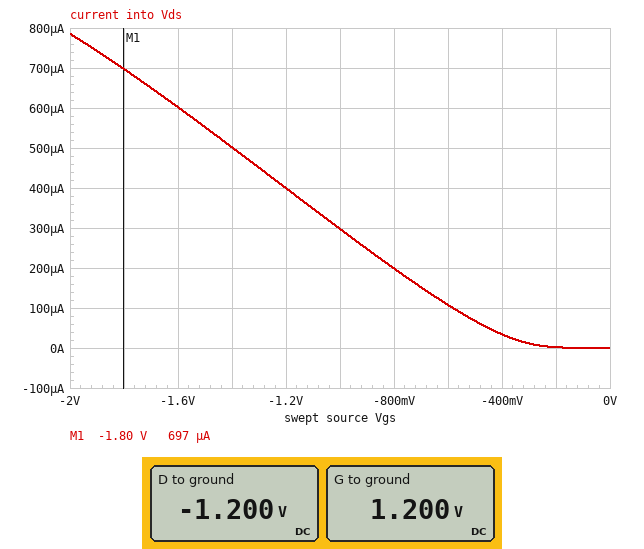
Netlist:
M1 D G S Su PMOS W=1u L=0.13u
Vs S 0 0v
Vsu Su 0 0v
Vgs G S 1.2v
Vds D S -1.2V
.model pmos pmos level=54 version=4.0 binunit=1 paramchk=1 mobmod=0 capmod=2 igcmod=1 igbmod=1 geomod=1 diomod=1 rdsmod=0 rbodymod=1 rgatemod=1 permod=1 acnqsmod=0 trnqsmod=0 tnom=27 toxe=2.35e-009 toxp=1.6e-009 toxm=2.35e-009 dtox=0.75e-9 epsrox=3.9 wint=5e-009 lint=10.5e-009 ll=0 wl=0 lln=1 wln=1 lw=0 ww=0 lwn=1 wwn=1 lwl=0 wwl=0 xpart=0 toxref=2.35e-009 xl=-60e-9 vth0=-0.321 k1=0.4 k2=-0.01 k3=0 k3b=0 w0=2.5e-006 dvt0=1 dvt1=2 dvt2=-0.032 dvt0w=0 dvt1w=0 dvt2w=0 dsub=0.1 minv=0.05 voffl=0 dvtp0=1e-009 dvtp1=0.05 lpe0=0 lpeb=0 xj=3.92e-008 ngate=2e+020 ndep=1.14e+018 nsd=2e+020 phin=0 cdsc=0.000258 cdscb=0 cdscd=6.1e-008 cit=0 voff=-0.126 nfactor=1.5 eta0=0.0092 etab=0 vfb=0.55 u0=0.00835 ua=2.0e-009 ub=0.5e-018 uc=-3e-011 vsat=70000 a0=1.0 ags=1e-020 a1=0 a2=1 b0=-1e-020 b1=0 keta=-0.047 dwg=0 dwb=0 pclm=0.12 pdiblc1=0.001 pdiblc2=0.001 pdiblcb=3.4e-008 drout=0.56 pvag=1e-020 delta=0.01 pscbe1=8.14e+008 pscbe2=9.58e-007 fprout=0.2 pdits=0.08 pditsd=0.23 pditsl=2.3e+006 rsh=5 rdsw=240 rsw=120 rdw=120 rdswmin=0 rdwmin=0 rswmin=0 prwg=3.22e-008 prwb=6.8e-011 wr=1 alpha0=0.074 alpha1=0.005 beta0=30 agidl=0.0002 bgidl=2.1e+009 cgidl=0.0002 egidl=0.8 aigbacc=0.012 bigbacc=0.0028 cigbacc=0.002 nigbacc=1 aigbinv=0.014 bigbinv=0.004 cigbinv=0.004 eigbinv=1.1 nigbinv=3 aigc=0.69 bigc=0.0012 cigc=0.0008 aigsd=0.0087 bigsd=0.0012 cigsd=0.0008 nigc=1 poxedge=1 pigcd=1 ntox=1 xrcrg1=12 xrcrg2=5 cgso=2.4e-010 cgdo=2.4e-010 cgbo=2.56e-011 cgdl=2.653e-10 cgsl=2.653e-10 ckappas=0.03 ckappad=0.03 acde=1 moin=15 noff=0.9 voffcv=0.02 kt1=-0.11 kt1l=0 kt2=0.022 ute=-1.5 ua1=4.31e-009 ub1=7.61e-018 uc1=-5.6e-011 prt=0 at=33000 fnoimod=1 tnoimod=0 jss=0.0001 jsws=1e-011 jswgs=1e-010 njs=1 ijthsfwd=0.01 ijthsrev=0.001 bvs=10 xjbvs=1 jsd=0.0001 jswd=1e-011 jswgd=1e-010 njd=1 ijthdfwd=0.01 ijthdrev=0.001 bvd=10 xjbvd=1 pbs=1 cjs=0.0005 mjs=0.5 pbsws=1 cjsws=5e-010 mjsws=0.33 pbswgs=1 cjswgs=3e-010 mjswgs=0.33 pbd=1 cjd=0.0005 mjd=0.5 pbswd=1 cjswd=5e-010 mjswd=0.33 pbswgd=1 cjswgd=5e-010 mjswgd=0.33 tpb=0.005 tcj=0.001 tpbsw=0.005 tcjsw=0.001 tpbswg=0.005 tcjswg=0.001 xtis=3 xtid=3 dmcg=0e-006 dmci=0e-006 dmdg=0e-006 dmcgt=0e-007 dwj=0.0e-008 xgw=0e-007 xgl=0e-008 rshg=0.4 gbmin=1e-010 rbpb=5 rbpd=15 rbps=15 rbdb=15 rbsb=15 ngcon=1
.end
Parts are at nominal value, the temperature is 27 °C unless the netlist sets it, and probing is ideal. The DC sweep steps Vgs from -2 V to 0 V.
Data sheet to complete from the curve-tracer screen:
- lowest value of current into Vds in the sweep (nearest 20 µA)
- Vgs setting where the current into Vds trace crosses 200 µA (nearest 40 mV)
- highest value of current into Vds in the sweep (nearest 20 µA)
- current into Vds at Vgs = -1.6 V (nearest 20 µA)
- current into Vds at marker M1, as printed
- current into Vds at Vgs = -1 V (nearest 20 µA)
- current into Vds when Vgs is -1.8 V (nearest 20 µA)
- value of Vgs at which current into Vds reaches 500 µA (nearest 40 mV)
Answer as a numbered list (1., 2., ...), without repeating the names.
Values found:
1. 0 A
2. -800 mV
3. 780 µA
4. 600 µA
5. 697 µA
6. 300 µA
7. 700 µA
8. -1.40 V
